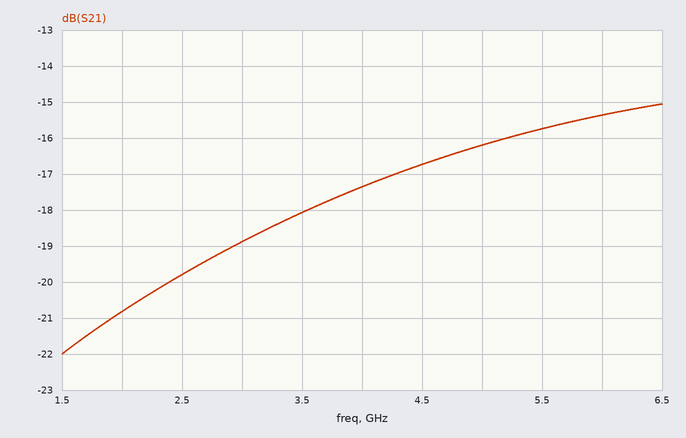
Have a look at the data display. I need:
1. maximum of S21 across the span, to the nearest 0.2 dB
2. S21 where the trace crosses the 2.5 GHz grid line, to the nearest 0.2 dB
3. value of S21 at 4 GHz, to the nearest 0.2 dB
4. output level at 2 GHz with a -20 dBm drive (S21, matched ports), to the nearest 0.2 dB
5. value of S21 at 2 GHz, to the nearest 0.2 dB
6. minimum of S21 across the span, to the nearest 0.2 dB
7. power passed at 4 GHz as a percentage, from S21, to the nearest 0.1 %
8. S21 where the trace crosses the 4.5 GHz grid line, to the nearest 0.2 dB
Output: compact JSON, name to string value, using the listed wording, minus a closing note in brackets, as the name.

{"maximum of S21 across the span, to the nearest 0.2 dB": "-15.0 dB", "S21 where the trace crosses the 2.5 GHz grid line, to the nearest 0.2 dB": "-19.8 dB", "value of S21 at 4 GHz, to the nearest 0.2 dB": "-17.4 dB", "output level at 2 GHz with a -20 dBm drive (S21, matched ports), to the nearest 0.2 dB": "-40.8 dBm", "value of S21 at 2 GHz, to the nearest 0.2 dB": "-20.8 dB", "minimum of S21 across the span, to the nearest 0.2 dB": "-22.0 dB", "power passed at 4 GHz as a percentage, from S21, to the nearest 0.1 %": "1.8 %", "S21 where the trace crosses the 4.5 GHz grid line, to the nearest 0.2 dB": "-16.8 dB"}
